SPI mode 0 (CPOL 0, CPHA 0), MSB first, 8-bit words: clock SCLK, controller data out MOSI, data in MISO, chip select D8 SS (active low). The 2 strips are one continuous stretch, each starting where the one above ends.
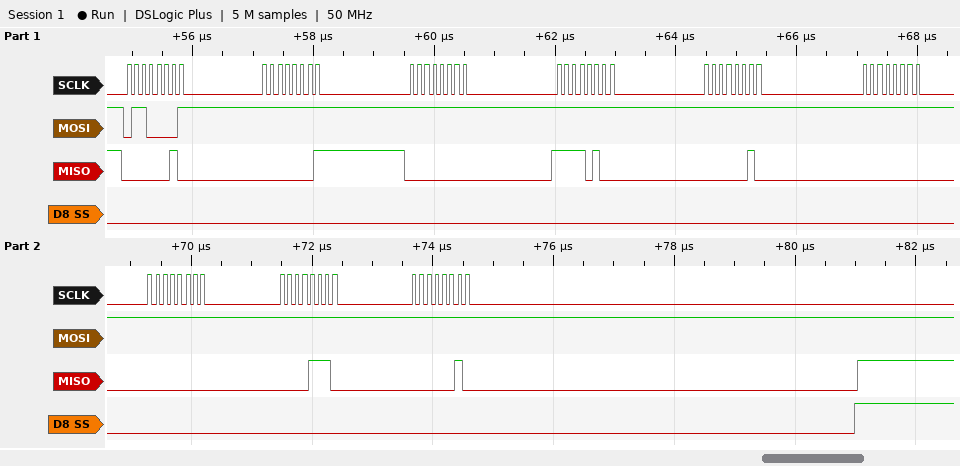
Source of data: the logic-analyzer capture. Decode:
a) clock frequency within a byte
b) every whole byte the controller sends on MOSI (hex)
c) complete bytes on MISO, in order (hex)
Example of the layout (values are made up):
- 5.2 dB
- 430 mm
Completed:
- 8 MHz
- 0x61 0xFF 0xFF 0xFF 0xFF 0xFF 0xFF 0xFF 0xFF
- 0x02 0x01 0x00 0xF4 0x02 0x00 0x00 0x0E 0x02
